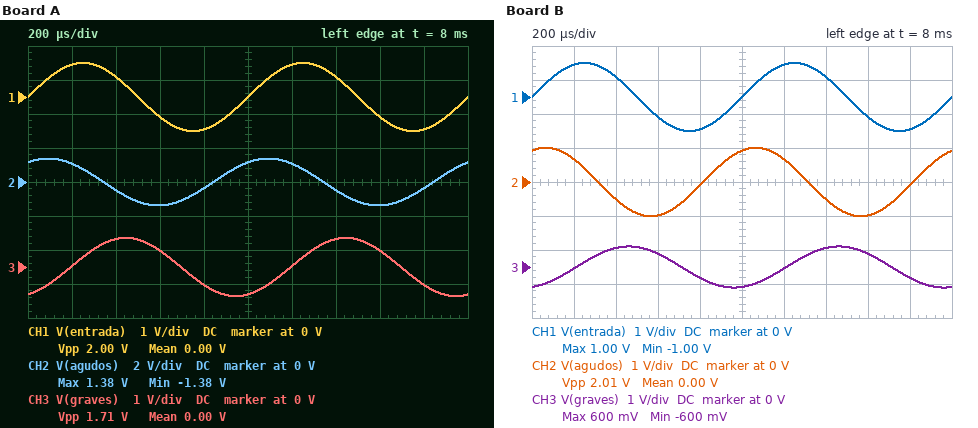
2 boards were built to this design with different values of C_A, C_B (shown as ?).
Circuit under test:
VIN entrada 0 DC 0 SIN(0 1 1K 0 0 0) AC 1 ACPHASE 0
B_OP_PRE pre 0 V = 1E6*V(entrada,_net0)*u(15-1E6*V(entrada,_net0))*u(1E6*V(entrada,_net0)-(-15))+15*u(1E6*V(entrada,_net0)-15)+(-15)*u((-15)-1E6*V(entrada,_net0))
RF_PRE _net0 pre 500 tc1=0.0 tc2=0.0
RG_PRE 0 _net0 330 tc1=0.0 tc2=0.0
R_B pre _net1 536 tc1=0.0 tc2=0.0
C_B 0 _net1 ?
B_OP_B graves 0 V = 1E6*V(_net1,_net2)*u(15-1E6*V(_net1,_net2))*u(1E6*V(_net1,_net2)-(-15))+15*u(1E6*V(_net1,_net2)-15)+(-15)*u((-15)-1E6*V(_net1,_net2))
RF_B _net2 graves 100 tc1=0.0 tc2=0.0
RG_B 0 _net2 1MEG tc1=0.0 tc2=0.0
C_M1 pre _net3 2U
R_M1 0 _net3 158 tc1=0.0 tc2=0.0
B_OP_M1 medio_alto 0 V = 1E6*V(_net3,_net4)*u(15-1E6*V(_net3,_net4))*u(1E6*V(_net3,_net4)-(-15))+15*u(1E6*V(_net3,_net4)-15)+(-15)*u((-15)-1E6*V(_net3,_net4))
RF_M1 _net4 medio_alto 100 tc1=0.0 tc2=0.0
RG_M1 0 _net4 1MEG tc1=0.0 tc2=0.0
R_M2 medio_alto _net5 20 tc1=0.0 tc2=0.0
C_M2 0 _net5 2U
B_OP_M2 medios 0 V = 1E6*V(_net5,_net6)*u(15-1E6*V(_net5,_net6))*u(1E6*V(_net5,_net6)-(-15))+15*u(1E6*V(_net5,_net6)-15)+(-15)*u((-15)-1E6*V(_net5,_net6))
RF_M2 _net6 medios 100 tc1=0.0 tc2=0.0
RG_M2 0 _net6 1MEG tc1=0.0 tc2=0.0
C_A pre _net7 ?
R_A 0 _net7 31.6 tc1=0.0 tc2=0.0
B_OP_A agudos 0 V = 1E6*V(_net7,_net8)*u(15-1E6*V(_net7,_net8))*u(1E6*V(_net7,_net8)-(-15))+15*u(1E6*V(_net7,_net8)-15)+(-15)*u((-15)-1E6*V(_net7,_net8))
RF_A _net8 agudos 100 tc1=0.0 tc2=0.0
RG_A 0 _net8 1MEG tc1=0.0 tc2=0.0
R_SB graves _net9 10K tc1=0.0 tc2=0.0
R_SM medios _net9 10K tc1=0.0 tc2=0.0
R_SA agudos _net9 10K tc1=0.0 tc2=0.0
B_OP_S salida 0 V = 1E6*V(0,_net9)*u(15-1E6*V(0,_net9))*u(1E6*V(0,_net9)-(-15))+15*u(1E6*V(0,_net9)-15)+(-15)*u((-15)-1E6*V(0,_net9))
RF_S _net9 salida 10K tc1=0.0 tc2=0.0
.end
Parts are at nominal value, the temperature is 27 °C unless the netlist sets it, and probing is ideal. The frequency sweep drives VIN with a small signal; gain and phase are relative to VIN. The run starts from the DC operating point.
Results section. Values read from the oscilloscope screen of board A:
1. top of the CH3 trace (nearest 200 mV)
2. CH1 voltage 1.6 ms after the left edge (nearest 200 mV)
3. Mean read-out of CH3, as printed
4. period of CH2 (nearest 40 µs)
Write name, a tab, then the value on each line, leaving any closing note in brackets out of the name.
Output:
top of the CH3 trace	800 mV
CH1 voltage 1.6 ms after the left edge	-600 mV
Mean read-out of CH3, as printed	0.00 V
period of CH2	1.00 ms
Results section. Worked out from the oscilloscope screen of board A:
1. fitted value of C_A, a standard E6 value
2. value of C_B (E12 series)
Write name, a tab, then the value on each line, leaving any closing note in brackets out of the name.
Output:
fitted value of C_A, a standard E6 value	3.3 µF
value of C_B	820 nF
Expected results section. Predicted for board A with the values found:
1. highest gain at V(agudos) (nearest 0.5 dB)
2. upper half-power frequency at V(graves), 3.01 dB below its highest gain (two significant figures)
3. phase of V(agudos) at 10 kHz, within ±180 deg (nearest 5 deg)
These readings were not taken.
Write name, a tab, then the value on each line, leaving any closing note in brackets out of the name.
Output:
highest gain at V(agudos)	8.0 dB
upper half-power frequency at V(graves), 3.01 dB below its highest gain	360 Hz
phase of V(agudos) at 10 kHz, within ±180 deg	10 deg
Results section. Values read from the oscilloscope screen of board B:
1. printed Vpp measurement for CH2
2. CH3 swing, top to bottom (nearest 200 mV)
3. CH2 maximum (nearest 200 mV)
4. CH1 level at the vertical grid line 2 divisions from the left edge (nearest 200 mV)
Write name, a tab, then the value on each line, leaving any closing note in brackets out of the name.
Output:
printed Vpp measurement for CH2	2.01 V
CH3 swing, top to bottom	1.2 V
CH2 maximum	1.0 V
CH1 level at the vertical grid line 2 divisions from the left edge	600 mV
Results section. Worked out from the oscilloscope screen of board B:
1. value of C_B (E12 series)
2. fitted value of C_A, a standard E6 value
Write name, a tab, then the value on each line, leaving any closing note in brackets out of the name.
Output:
value of C_B	1.2 µF
fitted value of C_A, a standard E6 value	2.2 µF
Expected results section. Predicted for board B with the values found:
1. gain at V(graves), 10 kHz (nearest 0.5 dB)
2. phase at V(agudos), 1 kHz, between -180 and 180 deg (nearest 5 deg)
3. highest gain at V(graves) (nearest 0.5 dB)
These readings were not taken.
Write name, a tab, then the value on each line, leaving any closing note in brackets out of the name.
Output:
gain at V(graves), 10 kHz	-24.0 dB
phase at V(agudos), 1 kHz, between -180 and 180 deg	65 deg
highest gain at V(graves)	8.0 dB
